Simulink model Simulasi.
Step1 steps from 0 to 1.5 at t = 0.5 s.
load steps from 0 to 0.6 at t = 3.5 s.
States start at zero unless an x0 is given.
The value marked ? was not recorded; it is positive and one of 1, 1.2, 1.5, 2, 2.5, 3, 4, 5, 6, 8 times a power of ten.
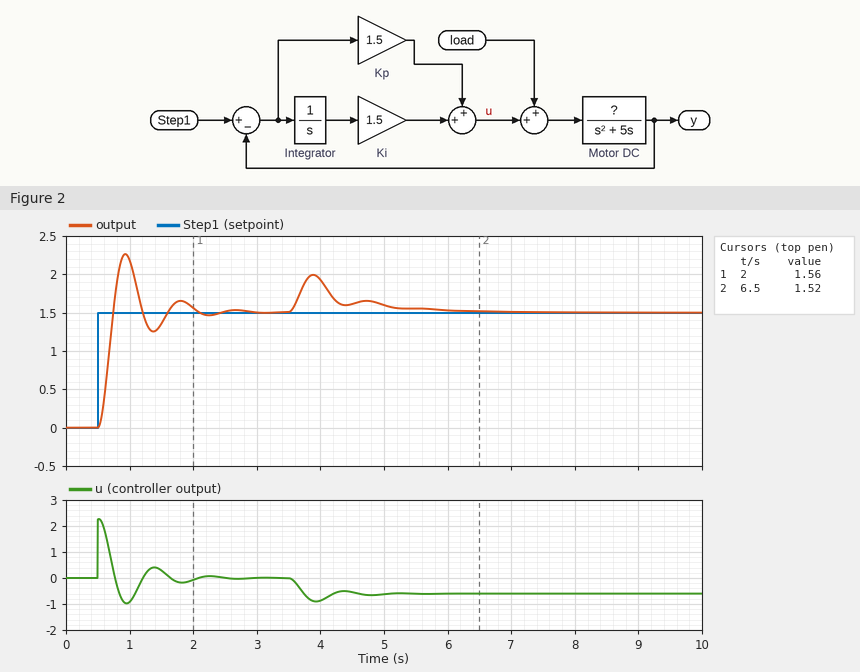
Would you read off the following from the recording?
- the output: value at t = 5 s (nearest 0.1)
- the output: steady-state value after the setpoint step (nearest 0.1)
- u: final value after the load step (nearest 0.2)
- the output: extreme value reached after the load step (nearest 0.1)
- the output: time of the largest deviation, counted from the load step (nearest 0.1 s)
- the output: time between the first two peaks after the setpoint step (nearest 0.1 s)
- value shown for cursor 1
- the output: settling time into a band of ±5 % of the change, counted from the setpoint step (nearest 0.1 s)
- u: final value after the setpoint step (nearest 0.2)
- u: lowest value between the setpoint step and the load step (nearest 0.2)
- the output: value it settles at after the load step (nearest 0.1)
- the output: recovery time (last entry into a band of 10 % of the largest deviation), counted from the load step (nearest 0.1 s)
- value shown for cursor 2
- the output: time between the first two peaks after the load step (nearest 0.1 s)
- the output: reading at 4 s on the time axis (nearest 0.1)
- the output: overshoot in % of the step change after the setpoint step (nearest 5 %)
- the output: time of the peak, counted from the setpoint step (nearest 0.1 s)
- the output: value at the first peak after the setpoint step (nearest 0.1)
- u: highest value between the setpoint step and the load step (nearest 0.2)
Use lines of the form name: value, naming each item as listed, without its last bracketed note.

the output: value at t = 5 s: 1.6
the output: steady-state value after the setpoint step: 1.5
u: final value after the load step: -0.6
the output: extreme value reached after the load step: 2.0
the output: time of the largest deviation, counted from the load step: 0.4 s
the output: time between the first two peaks after the setpoint step: 0.9 s
value shown for cursor 1: 1.56
the output: settling time into a band of ±5 % of the change, counted from the setpoint step: 1.5 s
u: final value after the setpoint step: 0.0
u: lowest value between the setpoint step and the load step: -1.0
the output: value it settles at after the load step: 1.5
the output: recovery time (last entry into a band of 10 % of the largest deviation), counted from the load step: 2.2 s
value shown for cursor 2: 1.52
the output: time between the first two peaks after the load step: 0.8 s
the output: reading at 4 s on the time axis: 1.9
the output: overshoot in % of the step change after the setpoint step: 50 %
the output: time of the peak, counted from the setpoint step: 0.4 s
the output: value at the first peak after the setpoint step: 2.3
u: highest value between the setpoint step and the load step: 2.2
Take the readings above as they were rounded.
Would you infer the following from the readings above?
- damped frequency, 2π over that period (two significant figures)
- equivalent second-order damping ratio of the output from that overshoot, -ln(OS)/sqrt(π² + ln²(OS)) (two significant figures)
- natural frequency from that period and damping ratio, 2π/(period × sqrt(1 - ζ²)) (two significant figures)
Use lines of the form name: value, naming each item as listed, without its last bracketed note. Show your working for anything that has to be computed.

damped frequency, 2π over that period: 2π / 0.9 = 7.0 rad/s
equivalent second-order damping ratio of the output from that overshoot, -ln(OS)/sqrt(π² + ln²(OS)): ln(0.5) = -0.693; 0.693 / sqrt(9.870 + 0.480) = 0.22
natural frequency from that period and damping ratio, 2π/(period × sqrt(1 - ζ²)): 2π / (0.9 × sqrt(1 - 0.22²)) = 7.2 rad/s
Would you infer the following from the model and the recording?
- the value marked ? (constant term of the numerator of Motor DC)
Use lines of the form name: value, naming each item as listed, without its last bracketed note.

the value marked ?: 40
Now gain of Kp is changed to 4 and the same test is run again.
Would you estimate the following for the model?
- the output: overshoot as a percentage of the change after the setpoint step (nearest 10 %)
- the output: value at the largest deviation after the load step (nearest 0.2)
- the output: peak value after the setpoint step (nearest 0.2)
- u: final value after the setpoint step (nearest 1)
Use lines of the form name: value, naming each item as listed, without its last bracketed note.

the output: overshoot as a percentage of the change after the setpoint step: 60 %
the output: value at the largest deviation after the load step: 1.8
the output: peak value after the setpoint step: 2.4
u: final value after the setpoint step: 0
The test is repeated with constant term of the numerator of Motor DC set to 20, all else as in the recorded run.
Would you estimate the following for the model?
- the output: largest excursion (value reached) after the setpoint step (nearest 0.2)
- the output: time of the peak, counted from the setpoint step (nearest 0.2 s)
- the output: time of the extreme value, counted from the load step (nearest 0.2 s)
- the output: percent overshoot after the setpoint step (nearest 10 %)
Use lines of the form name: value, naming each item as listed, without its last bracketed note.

the output: largest excursion (value reached) after the setpoint step: 2.2
the output: time of the peak, counted from the setpoint step: 0.6 s
the output: time of the extreme value, counted from the load step: 0.6 s
the output: percent overshoot after the setpoint step: 40 %
